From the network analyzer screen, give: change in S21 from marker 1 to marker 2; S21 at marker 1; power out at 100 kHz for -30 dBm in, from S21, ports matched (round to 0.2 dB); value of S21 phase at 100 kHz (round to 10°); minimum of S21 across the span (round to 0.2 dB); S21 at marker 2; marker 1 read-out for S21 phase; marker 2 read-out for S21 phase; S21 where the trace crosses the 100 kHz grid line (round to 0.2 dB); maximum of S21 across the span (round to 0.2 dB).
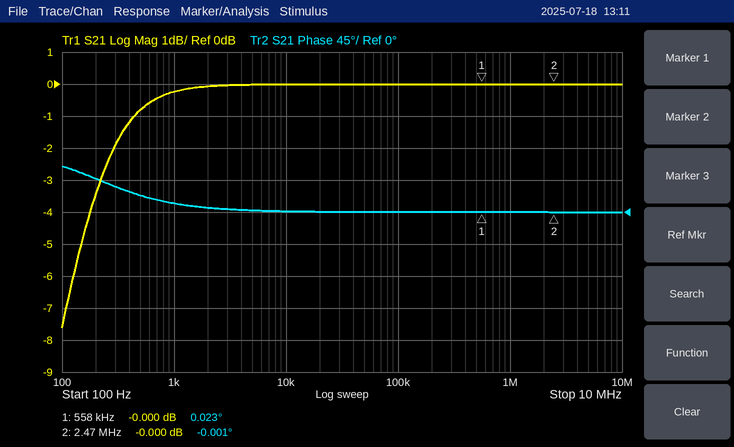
0.000 dB
-0.000 dB
-30.0 dBm
0°
-7.6 dB
-0.000 dB
0.023°
-0.001°
0.0 dB
0.0 dB
